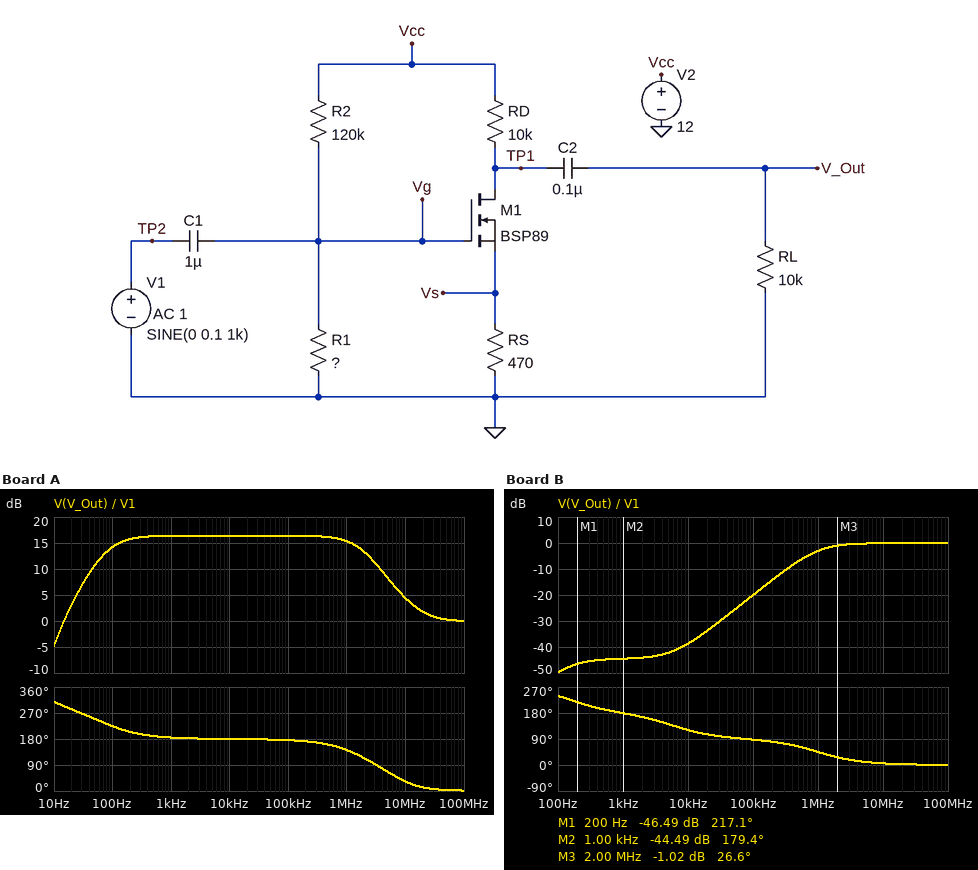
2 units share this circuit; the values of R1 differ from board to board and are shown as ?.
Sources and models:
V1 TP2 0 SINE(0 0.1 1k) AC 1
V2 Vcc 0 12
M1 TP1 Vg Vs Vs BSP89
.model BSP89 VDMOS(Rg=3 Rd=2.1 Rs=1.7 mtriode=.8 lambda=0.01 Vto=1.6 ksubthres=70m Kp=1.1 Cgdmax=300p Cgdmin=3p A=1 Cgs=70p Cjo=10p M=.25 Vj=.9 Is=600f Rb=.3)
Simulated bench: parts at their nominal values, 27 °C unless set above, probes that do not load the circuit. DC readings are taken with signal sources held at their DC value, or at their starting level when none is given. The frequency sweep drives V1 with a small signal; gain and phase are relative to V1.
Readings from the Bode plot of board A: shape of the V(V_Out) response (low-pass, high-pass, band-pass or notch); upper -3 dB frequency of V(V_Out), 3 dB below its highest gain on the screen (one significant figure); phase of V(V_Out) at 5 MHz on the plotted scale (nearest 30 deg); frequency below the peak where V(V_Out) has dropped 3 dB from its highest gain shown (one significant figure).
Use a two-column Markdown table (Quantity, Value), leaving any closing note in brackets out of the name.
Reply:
| Quantity | Value |
|---|---|
| shape of the V(V_Out) response | band-pass |
| upper -3 dB frequency of V(V_Out), 3 dB below its highest gain on the screen | 2 MHz |
| phase of V(V_Out) at 5 MHz on the plotted scale | 60 deg |
| frequency below the peak where V(V_Out) has dropped 3 dB from its highest gain shown | 80 Hz |
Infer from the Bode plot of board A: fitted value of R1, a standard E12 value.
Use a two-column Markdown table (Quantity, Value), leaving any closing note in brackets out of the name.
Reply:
| Quantity | Value |
|---|---|
| fitted value of R1, a standard E12 value | 18 kΩ |
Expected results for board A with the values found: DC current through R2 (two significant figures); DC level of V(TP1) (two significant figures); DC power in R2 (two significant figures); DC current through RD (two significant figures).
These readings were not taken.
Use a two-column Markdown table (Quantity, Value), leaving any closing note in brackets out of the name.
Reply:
| Quantity | Value |
|---|---|
| DC current through R2 | 87 µA |
| DC level of V(TP1) | 11 V |
| DC power in R2 | 910 µW |
| DC current through RD | 140 µA |
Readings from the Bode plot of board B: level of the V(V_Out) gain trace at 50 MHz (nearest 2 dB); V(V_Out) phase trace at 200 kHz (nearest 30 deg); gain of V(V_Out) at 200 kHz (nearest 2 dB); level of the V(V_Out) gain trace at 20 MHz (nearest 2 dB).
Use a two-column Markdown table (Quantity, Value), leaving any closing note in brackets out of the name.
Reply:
| Quantity | Value |
|---|---|
| level of the V(V_Out) gain trace at 50 MHz | 0 dB |
| V(V_Out) phase trace at 200 kHz | 90 deg |
| gain of V(V_Out) at 200 kHz | -14 dB |
| level of the V(V_Out) gain trace at 20 MHz | 0 dB |
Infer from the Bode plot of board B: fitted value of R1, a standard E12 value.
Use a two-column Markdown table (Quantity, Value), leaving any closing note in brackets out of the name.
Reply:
| Quantity | Value |
|---|---|
| fitted value of R1, a standard E12 value | 33 kΩ |
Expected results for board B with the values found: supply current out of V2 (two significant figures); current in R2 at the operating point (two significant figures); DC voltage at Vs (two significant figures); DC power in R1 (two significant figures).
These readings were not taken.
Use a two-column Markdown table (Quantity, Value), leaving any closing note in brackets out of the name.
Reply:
| Quantity | Value |
|---|---|
| supply current out of V2 | 1.2 mA |
| current in R2 at the operating point | 78 µA |
| DC voltage at Vs | 540 mV |
| DC power in R1 | 200 µW |
